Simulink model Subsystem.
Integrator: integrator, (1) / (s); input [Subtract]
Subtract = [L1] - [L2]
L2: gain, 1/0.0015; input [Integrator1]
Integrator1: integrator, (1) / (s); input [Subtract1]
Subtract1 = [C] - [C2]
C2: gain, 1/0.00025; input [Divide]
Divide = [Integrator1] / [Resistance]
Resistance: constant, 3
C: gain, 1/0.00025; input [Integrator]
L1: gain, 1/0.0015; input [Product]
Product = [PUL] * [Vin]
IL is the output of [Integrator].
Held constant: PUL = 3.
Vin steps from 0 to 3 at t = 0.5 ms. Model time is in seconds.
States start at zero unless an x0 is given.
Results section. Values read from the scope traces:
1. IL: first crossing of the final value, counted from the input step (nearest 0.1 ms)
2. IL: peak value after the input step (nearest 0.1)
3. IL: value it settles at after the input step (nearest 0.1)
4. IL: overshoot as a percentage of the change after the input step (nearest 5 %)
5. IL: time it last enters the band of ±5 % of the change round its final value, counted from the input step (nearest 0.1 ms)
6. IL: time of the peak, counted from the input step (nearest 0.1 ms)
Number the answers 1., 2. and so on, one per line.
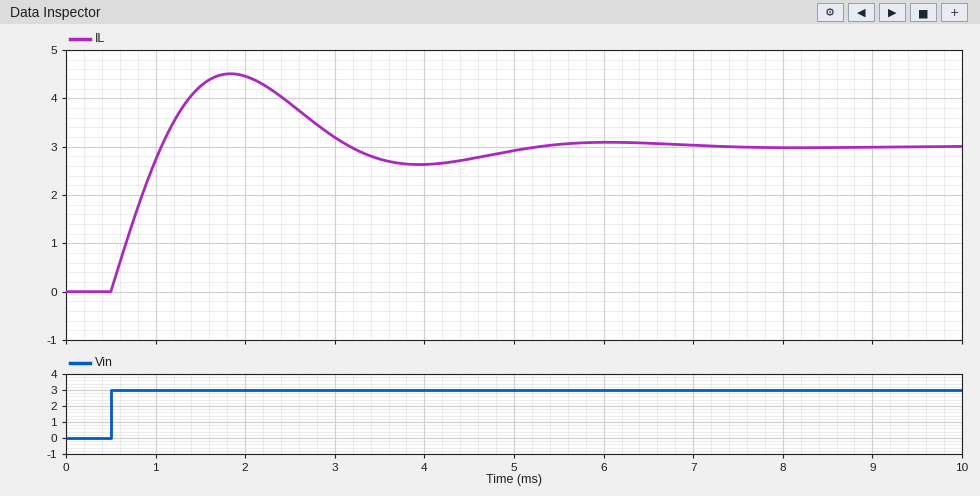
1. 0.6 ms
2. 4.5
3. 3.0
4. 50 %
5. 4.3 ms
6. 1.3 ms
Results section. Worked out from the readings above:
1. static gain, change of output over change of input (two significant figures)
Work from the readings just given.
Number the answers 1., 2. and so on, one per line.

1. 1.0
